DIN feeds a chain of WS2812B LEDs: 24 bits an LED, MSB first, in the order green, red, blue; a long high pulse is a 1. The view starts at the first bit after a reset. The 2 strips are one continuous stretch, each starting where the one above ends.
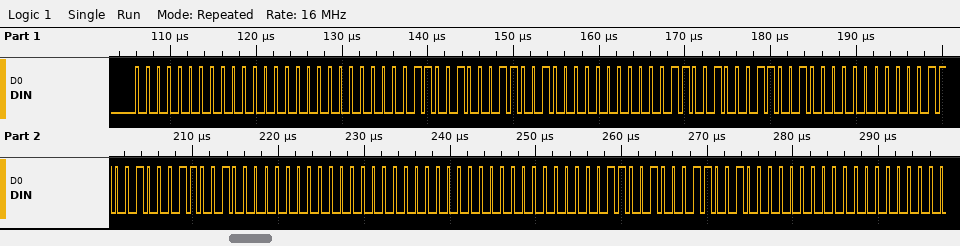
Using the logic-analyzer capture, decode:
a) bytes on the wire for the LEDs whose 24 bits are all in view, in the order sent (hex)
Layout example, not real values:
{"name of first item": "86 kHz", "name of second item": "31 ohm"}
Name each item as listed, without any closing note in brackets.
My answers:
{"bytes on the wire for the LEDs whose 24 bits are all in view, in the order sent": "00 00 00 32 32 00 32 32 00 32 32 00 00 00 00 32 32 00"}
